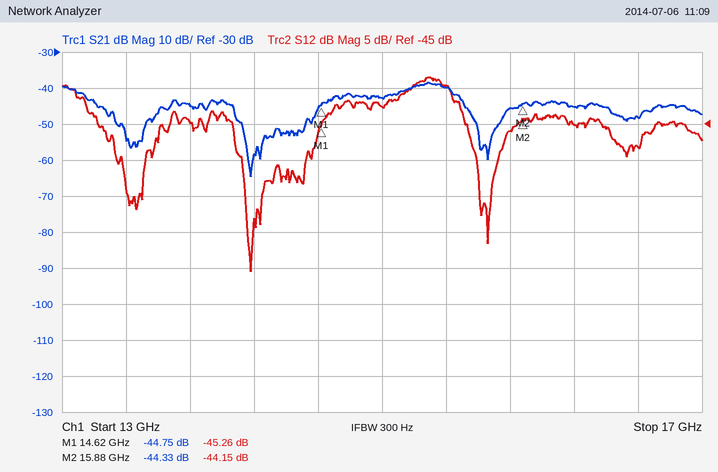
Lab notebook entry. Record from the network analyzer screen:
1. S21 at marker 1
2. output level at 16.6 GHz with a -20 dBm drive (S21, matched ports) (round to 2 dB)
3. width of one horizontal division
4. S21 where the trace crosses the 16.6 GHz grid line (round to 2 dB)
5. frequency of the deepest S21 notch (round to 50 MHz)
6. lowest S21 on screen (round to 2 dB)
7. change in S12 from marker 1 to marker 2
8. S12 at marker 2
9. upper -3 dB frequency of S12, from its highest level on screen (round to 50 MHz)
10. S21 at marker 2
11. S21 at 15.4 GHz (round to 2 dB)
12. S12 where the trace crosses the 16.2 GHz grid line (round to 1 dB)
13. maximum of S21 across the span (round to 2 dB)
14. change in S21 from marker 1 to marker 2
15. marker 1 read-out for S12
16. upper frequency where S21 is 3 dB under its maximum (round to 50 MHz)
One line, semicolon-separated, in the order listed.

-44.75 dB; -68 dBm; 400 MHz; -48 dB; 14.20 GHz; -64 dB; 1.11 dB; -44.15 dB; 15.45 GHz; -44.33 dB; -40 dB; -45 dB; -38 dB; 0.42 dB; -45.26 dB; 15.45 GHz
